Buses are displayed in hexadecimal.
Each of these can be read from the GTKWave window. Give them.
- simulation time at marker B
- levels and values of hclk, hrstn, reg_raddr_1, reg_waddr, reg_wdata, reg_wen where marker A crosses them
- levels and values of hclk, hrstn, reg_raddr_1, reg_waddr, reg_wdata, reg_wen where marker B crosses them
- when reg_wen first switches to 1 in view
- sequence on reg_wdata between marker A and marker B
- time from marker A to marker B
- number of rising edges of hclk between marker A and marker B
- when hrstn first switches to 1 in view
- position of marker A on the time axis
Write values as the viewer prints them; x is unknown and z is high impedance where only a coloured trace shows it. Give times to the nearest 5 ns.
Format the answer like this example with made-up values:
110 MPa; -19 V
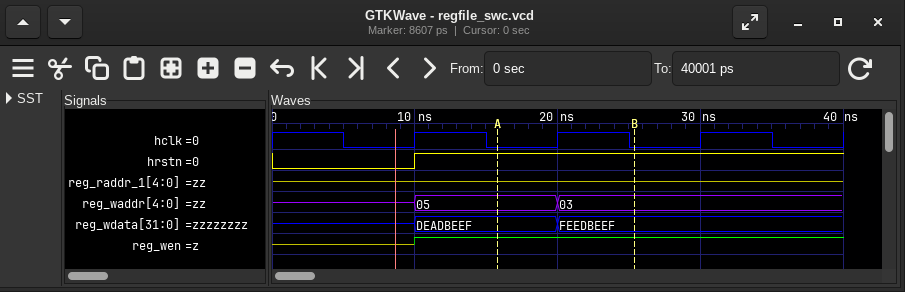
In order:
25 ns; hclk=0, hrstn=1, reg_raddr_1=z, reg_waddr=05, reg_wdata=DEADBEEF, reg_wen=1; hclk=0, hrstn=1, reg_raddr_1=z, reg_waddr=03, reg_wdata=FEEDBEEF, reg_wen=1; 10 ns; DEADBEEF, FEEDBEEF; 10 ns; 1; 10 ns; 15 ns
